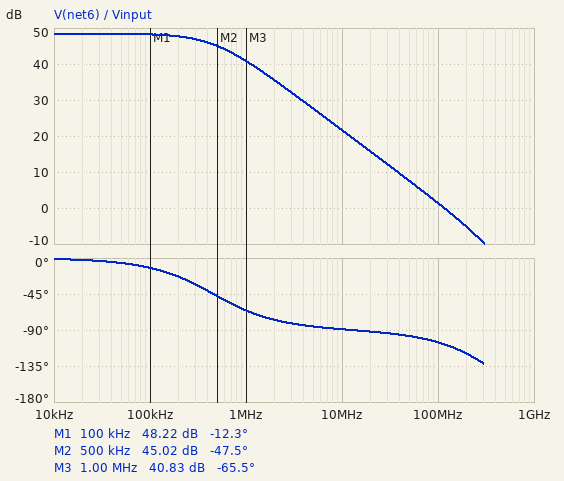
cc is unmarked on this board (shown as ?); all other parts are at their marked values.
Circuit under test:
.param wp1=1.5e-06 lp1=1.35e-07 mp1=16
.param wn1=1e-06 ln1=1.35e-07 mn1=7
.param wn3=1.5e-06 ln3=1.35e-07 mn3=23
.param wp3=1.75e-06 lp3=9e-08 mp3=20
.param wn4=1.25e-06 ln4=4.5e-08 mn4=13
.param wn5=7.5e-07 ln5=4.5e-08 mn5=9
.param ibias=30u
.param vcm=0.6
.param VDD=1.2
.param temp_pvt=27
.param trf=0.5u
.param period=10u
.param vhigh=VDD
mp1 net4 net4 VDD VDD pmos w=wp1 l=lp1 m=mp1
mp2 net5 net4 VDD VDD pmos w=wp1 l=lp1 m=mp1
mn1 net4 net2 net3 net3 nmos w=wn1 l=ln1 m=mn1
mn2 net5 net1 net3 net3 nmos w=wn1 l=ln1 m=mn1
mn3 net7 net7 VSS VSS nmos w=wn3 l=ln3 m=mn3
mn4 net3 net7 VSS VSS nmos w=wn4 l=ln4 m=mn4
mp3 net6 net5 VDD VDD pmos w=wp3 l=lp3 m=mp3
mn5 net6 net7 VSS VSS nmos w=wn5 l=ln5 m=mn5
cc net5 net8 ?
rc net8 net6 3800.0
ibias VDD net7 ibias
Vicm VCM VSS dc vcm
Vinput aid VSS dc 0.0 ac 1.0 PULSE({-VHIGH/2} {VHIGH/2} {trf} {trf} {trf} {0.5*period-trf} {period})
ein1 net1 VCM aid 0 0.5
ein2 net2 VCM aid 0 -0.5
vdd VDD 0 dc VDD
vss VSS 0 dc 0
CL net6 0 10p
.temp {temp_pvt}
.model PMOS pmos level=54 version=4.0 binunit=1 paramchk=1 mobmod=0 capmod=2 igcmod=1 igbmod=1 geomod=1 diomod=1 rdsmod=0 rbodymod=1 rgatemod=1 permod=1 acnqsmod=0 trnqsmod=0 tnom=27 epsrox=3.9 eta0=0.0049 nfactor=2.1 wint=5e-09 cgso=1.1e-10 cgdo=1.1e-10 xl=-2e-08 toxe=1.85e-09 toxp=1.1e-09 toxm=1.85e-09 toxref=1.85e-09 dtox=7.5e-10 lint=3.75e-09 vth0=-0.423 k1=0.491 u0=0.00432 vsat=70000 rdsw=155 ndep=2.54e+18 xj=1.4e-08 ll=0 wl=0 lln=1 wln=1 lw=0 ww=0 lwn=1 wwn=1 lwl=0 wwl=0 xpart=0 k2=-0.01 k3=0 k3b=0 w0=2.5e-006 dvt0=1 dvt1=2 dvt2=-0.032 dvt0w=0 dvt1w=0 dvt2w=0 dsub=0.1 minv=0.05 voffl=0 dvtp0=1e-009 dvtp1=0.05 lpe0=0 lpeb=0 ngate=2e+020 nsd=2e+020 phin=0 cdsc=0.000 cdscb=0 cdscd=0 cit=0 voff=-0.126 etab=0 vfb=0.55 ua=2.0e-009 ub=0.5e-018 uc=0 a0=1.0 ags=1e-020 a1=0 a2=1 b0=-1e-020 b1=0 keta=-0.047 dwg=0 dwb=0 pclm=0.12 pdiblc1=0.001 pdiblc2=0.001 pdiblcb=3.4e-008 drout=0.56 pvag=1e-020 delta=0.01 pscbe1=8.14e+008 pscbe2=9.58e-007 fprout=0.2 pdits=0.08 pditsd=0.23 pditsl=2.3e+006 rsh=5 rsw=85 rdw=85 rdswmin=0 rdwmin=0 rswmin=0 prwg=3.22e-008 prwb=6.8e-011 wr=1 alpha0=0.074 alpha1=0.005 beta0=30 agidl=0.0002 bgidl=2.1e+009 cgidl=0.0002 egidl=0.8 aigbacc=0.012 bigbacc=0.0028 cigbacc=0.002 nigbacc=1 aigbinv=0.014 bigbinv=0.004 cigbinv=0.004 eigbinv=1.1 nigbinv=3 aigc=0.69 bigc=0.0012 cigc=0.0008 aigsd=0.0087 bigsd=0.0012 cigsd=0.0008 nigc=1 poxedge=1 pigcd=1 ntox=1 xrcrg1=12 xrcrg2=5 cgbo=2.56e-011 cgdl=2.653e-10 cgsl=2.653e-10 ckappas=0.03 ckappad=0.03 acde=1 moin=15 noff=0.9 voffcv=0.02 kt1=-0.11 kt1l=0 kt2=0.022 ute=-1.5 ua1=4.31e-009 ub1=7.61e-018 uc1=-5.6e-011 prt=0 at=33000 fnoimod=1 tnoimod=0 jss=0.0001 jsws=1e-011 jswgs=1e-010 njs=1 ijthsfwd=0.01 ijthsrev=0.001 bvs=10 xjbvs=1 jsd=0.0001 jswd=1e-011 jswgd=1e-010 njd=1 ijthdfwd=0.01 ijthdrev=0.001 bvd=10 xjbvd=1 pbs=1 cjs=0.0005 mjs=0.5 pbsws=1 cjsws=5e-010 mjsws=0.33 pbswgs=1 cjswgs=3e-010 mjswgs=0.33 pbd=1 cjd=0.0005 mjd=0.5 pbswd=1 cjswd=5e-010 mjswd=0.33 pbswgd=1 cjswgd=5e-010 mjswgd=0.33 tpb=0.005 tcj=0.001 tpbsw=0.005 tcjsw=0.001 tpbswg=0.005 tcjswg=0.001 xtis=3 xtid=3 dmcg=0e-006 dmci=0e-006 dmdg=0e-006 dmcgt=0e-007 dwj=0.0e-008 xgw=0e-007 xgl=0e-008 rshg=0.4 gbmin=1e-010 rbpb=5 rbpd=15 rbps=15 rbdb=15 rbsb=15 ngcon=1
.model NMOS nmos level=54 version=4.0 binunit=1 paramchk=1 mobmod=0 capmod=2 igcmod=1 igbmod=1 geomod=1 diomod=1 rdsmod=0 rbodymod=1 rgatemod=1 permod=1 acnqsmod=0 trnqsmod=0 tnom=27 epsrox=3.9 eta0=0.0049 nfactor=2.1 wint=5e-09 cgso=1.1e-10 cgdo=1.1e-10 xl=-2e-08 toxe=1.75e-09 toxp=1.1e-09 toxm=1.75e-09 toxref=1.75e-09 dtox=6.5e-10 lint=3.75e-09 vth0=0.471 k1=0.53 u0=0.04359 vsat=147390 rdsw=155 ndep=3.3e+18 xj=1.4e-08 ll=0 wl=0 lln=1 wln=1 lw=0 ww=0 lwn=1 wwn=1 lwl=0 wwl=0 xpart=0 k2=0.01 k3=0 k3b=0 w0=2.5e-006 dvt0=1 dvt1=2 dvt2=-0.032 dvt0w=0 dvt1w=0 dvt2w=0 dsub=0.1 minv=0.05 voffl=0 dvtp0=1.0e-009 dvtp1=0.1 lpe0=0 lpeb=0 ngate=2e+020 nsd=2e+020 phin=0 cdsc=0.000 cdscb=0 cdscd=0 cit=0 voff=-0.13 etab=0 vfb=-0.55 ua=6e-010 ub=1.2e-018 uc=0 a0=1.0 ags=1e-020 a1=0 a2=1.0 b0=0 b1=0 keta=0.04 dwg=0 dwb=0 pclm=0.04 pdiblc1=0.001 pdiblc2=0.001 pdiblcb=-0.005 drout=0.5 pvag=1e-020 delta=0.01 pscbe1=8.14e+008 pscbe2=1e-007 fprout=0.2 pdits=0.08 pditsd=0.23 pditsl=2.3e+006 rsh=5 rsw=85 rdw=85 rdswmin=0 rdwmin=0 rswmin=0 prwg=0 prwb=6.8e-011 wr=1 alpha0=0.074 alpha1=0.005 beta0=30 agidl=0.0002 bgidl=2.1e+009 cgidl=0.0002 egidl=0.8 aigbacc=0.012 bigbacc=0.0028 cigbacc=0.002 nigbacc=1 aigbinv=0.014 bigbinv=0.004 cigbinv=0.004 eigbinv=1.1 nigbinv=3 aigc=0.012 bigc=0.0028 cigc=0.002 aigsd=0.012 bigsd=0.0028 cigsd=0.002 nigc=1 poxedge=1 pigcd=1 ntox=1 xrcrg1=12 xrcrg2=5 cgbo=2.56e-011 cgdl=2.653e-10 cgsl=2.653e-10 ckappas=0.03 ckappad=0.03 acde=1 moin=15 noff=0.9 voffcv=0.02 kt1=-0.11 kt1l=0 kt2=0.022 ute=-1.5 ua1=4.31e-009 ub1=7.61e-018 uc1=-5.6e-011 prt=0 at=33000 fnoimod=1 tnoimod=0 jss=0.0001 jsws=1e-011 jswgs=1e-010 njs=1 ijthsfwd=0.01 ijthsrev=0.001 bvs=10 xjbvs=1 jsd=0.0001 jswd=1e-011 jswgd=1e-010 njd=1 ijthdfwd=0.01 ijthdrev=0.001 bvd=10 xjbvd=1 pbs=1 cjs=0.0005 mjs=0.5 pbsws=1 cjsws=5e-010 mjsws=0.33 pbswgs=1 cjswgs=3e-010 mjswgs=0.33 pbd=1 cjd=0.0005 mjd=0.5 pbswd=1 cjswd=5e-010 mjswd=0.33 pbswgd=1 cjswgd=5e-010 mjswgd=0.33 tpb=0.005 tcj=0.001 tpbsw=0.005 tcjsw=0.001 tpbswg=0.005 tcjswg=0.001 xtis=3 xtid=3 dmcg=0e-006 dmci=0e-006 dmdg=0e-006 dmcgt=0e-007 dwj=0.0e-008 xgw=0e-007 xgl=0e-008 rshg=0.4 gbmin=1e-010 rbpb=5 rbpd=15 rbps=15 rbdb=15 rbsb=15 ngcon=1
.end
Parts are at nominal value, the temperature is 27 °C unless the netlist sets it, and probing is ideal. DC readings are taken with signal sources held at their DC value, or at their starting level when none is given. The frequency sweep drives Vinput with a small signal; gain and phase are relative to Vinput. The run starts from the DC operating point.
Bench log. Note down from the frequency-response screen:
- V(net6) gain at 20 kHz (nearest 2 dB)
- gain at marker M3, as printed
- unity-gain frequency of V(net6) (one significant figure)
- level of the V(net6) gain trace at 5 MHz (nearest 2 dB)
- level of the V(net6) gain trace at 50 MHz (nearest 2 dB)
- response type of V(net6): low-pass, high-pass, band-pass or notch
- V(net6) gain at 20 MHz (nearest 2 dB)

48 dB
40.83 dB
100 MHz
28 dB
8 dB
low-pass
16 dB
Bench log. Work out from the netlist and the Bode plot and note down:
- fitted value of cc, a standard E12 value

1 pF
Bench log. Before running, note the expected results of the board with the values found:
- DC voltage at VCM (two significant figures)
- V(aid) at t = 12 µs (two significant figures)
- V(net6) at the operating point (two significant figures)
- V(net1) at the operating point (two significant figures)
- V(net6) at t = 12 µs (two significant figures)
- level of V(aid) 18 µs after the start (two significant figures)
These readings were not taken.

600 mV
600 mV
520 mV
600 mV
1.1 V
-600 mV
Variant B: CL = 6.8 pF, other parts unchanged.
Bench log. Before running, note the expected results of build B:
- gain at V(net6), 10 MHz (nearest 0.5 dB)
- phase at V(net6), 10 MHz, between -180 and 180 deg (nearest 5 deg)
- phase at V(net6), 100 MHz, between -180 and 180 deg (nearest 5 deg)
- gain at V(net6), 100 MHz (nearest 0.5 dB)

22.0 dB
-85 deg
-95 deg
4.0 dB
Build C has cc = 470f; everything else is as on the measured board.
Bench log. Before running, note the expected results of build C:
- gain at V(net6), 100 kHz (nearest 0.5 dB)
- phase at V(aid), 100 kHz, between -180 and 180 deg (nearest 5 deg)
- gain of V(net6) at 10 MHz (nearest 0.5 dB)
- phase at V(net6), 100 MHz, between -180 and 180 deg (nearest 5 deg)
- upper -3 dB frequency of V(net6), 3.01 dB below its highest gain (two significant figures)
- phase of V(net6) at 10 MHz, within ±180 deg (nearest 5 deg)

48.5 dB
0 deg
27.5 dB
-125 deg
910 kHz
-95 deg
